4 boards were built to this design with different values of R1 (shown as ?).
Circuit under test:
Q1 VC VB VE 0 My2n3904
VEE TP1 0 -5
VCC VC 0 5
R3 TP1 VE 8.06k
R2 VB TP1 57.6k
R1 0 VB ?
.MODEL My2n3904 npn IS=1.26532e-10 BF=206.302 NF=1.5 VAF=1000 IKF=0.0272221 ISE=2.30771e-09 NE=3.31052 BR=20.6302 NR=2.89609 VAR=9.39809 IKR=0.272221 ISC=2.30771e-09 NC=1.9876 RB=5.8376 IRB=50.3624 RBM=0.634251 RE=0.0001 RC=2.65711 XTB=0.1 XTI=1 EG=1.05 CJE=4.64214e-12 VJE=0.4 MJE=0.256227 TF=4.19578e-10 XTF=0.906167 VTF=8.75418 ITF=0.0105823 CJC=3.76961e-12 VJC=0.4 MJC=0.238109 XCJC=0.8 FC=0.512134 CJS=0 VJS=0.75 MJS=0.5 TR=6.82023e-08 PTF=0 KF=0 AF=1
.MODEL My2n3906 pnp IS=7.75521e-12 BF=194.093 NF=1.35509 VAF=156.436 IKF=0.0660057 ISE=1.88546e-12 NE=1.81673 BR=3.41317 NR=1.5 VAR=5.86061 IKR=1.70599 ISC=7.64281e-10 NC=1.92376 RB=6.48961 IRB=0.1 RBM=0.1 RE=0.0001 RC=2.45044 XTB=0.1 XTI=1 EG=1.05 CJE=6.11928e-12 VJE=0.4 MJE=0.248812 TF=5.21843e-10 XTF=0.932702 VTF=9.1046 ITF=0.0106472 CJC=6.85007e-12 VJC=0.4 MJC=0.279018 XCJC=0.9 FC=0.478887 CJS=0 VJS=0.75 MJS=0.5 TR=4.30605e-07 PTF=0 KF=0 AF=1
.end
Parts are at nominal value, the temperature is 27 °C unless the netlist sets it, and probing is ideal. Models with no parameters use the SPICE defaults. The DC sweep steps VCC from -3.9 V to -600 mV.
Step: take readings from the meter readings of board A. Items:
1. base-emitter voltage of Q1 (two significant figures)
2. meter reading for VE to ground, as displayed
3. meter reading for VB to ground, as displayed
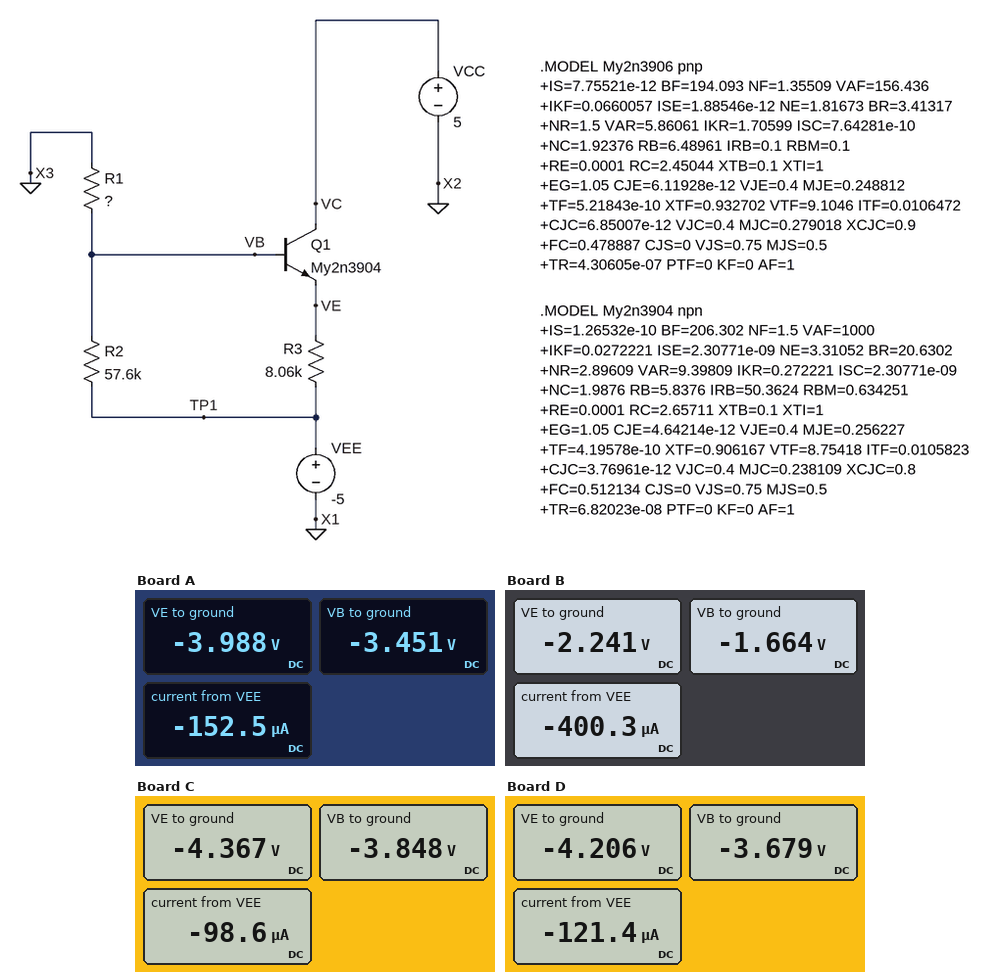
540 mV
-3.988 V
-3.451 V
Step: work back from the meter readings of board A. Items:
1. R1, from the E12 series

120 kΩ
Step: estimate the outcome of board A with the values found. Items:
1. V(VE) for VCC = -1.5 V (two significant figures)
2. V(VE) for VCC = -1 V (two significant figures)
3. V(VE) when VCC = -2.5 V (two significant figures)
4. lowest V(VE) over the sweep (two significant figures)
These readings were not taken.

-4.0 V
-4.0 V
-4.0 V
-4.1 V
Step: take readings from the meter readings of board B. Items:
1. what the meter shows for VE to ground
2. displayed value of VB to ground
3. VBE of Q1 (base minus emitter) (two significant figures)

-2.241 V
-1.664 V
580 mV
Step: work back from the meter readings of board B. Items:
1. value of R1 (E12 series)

27 kΩ
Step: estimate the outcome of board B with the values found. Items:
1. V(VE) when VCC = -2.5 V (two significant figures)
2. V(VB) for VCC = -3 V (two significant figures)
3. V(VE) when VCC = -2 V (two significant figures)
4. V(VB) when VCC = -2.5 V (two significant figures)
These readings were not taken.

-2.6 V
-2.5 V
-2.3 V
-2.0 V
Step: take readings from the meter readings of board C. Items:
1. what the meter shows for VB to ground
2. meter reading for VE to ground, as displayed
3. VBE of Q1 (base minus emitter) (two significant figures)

-3.848 V
-4.367 V
520 mV
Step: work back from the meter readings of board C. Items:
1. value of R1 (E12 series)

180 kΩ
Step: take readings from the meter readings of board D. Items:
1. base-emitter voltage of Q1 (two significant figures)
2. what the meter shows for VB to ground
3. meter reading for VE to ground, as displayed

530 mV
-3.679 V
-4.206 V
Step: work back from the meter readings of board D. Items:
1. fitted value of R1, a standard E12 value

150 kΩ
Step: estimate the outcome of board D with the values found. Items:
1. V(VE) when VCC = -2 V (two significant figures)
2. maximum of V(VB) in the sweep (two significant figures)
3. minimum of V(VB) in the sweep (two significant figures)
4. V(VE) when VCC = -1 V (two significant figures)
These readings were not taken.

-4.2 V
-3.7 V
-3.7 V
-4.2 V
